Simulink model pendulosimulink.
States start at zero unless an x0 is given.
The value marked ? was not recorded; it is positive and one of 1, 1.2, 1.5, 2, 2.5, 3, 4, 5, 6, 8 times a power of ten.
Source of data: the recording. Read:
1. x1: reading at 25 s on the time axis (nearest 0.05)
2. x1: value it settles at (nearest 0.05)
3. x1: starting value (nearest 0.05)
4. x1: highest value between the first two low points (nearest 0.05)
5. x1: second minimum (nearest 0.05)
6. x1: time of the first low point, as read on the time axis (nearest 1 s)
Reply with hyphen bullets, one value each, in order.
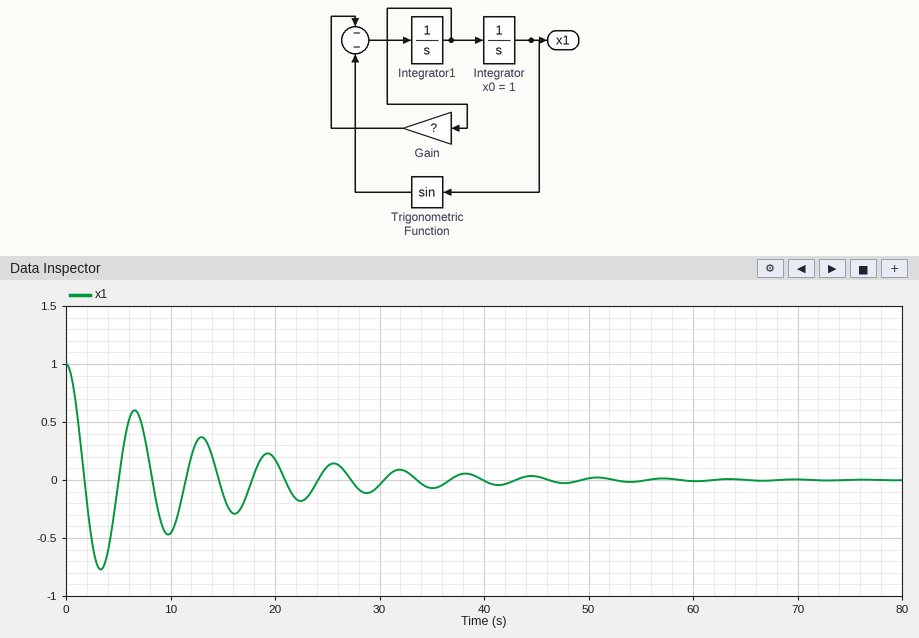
- 0.10
- 0.00
- 1.00
- 0.60
- -0.45
- 3 s
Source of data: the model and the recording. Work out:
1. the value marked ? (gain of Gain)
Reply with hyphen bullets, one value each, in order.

- 0.15
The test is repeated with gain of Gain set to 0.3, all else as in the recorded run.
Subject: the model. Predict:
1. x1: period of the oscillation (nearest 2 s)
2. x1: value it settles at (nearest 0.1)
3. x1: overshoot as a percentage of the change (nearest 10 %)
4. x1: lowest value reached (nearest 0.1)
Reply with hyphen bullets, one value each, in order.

- 6 s
- 0.0
- 60 %
- -0.6
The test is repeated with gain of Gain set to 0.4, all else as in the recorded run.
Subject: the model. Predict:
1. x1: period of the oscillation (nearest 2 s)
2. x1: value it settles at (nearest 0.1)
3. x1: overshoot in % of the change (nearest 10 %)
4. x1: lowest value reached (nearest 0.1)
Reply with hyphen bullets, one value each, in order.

- 6 s
- 0.0
- 50 %
- -0.5
